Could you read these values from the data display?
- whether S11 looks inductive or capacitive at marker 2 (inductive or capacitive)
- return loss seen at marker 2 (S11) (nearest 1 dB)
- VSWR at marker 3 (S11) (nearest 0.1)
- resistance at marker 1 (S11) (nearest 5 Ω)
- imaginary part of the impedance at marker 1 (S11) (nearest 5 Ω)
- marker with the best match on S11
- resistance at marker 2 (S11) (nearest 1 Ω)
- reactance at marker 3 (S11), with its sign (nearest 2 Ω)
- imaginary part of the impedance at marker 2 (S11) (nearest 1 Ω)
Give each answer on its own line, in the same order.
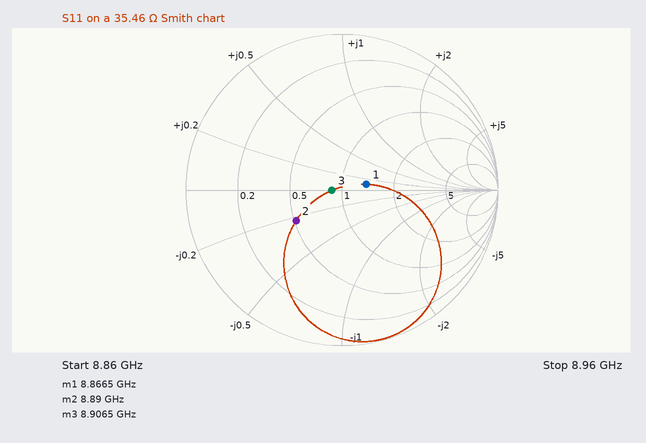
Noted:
capacitive
9 dB
1.1
50 Ω
+5 Ω
marker 3
18 Ω
0 Ω
-8 Ω
